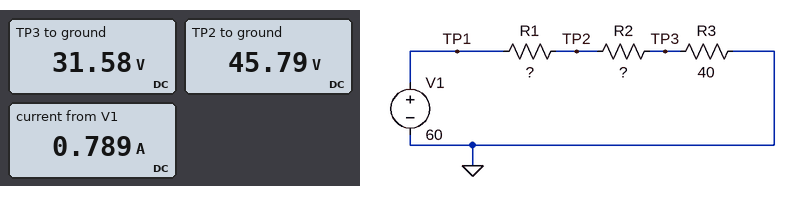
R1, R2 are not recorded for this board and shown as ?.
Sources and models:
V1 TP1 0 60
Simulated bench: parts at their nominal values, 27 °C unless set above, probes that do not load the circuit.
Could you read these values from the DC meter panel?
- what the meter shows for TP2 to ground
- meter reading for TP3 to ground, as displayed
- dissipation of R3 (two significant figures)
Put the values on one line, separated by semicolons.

45.79 V; 31.58 V; 25 W
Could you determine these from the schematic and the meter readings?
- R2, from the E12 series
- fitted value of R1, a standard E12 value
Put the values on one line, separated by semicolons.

18 Ω; 18 Ω
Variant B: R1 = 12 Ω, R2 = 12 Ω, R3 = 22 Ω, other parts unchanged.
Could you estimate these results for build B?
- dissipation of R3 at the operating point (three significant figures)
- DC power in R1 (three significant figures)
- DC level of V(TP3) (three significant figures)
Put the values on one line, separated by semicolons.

37.4 W; 20.4 W; 28.7 V
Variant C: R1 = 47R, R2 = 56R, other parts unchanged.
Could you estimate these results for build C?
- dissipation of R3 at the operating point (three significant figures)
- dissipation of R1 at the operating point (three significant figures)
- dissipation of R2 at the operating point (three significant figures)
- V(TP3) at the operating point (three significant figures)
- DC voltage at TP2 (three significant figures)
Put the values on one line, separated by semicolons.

7.04 W; 8.27 W; 9.86 W; 16.8 V; 40.3 V
